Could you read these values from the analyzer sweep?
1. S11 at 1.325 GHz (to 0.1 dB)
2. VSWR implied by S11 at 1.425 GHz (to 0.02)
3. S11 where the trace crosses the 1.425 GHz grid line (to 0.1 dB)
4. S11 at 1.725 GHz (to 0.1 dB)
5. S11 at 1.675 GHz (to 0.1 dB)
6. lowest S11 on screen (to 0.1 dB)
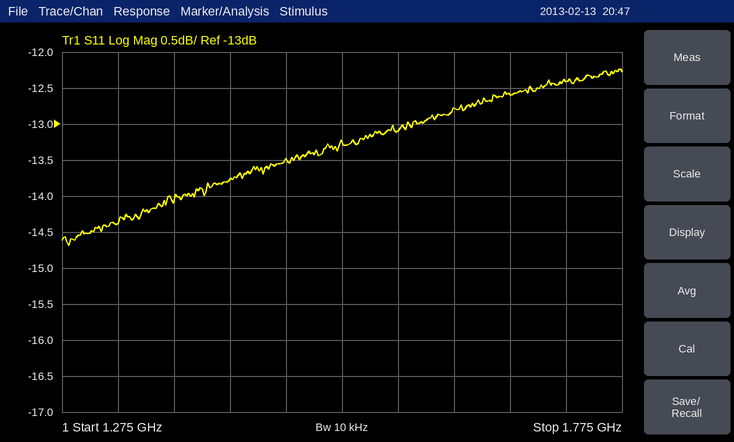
-14.4 dB
1.52
-13.8 dB
-12.4 dB
-12.6 dB
-14.7 dB
